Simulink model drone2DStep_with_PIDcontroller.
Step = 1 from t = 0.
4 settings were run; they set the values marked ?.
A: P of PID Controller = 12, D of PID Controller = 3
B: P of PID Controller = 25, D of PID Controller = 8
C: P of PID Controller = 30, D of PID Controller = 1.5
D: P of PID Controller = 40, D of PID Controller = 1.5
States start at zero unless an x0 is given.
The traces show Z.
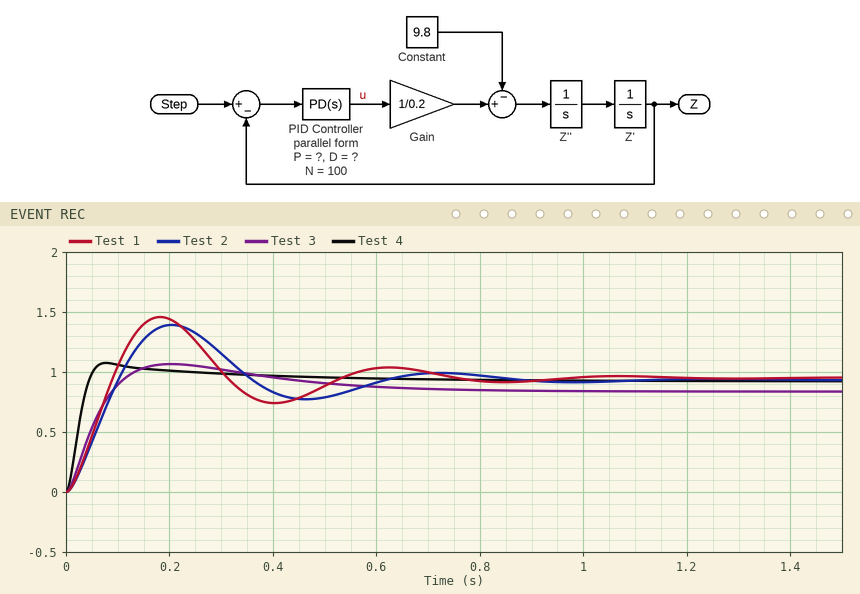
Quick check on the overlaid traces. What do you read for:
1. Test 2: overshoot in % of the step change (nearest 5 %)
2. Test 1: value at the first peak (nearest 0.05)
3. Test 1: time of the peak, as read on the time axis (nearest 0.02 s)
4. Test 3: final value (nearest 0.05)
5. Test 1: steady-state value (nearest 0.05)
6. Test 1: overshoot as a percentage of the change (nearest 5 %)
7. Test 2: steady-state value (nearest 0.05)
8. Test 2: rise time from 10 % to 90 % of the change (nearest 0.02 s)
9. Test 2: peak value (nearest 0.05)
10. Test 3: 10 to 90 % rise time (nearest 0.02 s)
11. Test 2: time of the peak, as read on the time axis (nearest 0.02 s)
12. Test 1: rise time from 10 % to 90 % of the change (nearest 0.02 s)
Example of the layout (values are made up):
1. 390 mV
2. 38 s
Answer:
1. 50 %
2. 1.45
3. 0.18 s
4. 0.85
5. 0.95
6. 55 %
7. 0.95
8. 0.08 s
9. 1.40
10. 0.06 s
11. 0.20 s
12. 0.06 s
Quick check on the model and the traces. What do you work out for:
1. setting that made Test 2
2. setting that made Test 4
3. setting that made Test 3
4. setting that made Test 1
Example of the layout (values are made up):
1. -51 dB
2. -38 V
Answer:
1. C
2. B
3. A
4. D
